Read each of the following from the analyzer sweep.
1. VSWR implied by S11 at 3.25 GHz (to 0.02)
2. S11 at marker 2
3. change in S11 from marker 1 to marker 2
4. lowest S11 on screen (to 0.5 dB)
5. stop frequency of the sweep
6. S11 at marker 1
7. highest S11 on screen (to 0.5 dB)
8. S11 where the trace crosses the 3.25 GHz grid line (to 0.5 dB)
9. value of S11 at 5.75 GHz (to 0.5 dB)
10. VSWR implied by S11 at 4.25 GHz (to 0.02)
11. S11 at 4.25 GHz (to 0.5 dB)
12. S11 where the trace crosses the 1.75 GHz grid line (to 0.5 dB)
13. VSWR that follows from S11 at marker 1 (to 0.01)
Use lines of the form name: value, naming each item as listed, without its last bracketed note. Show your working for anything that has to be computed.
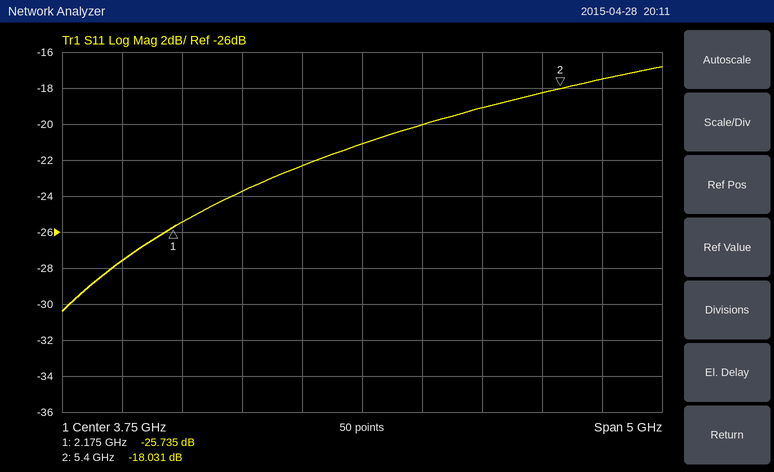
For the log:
VSWR implied by S11 at 3.25 GHz: |Γ| = 10^(-22.5/20) = 0.0750; VSWR = (1 + 0.0750)/(1 − 0.0750) ≈ 1.16
S11 at marker 2: -18.031 dB
change in S11 from marker 1 to marker 2: -18.031 − (-25.735) = 7.704 dB
lowest S11 on screen: -30.5 dB
stop frequency of the sweep: 6.25 GHz
S11 at marker 1: -25.735 dB
highest S11 on screen: -17.0 dB
S11 where the trace crosses the 3.25 GHz grid line: -22.5 dB
value of S11 at 5.75 GHz: -17.5 dB
VSWR implied by S11 at 4.25 GHz: |Γ| = 10^(-20/20) = 0.1000; VSWR = (1 + 0.1000)/(1 − 0.1000) ≈ 1.22
S11 at 4.25 GHz: -20.0 dB
S11 where the trace crosses the 1.75 GHz grid line: -27.5 dB
VSWR that follows from S11 at marker 1: (1 + 0.0517)/(1 − 0.0517) ≈ 1.11
